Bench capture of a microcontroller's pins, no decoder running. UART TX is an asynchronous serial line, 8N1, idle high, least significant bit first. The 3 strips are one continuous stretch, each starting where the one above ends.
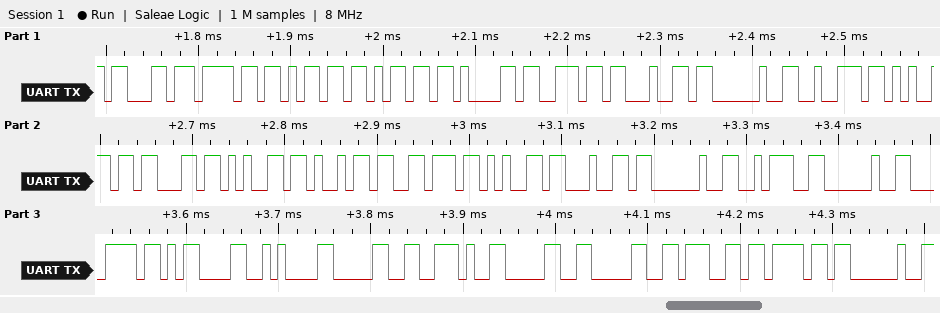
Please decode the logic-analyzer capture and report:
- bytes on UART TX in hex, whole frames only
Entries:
63 6F 6D 6D 61 6E 64 20 72 65 63 65 69 76 65 64 20 3A 20 78 0D 0A 30 2E 30 30 67 6F 20
